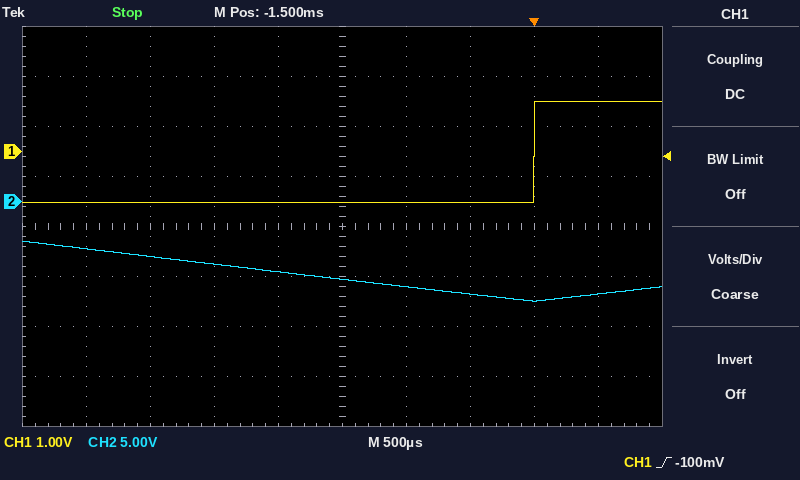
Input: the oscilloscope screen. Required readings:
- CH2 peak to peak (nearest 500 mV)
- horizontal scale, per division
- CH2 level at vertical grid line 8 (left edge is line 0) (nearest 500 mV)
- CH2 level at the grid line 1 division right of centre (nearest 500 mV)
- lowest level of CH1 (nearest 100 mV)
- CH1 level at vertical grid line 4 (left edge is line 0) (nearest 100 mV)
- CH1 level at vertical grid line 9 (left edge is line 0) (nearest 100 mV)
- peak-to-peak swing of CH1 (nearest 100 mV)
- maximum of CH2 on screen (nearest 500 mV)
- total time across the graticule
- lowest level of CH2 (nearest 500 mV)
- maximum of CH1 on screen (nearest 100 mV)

6.0 V
500 µs
-10.0 V
-8.5 V
-1.0 V
-1.0 V
1.0 V
2.0 V
-4.0 V
5 ms
-10.0 V
1.0 V
